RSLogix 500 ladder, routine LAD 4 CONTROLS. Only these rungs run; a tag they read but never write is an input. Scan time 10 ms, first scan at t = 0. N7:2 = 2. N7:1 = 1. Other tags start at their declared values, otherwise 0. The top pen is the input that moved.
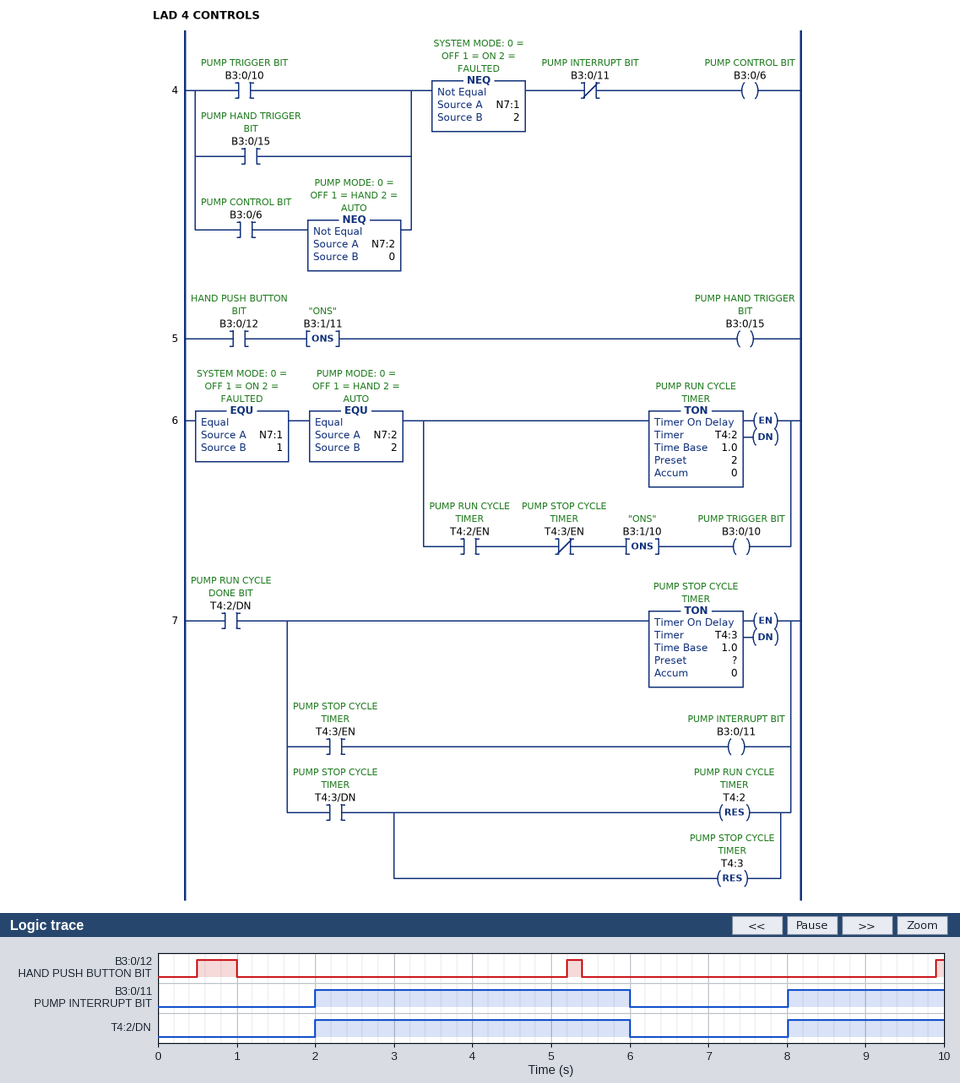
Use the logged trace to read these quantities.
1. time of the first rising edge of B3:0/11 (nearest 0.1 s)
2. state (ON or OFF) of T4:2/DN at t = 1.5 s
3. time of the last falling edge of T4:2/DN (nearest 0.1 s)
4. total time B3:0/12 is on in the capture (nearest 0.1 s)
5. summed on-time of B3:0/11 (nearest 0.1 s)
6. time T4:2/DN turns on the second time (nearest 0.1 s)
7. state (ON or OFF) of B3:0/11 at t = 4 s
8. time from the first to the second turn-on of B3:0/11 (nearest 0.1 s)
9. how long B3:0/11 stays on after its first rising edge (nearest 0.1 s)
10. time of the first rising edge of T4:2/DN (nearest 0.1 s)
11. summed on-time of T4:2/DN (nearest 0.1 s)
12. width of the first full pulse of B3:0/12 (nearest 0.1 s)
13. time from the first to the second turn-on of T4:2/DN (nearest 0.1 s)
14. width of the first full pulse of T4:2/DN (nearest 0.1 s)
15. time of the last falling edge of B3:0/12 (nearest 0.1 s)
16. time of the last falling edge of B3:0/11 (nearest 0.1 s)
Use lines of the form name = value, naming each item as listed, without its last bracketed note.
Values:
time of the first rising edge of B3:0/11 = 2.0 s
state (ON or OFF) of T4:2/DN at t = 1.5 s = OFF
time of the last falling edge of T4:2/DN = 6.0 s
total time B3:0/12 is on in the capture = 0.8 s
summed on-time of B3:0/11 = 6.0 s
time T4:2/DN turns on the second time = 8.0 s
state (ON or OFF) of B3:0/11 at t = 4 s = ON
time from the first to the second turn-on of B3:0/11 = 6.0 s
how long B3:0/11 stays on after its first rising edge = 4.0 s
time of the first rising edge of T4:2/DN = 2.0 s
summed on-time of T4:2/DN = 6.0 s
width of the first full pulse of B3:0/12 = 0.5 s
time from the first to the second turn-on of T4:2/DN = 6.0 s
width of the first full pulse of T4:2/DN = 4.0 s
time of the last falling edge of B3:0/12 = 5.4 s
time of the last falling edge of B3:0/11 = 6.0 s
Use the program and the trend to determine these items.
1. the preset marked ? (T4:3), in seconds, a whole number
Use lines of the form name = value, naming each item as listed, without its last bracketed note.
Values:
the preset marked ? (T4:3), in seconds, a whole number = 4 s
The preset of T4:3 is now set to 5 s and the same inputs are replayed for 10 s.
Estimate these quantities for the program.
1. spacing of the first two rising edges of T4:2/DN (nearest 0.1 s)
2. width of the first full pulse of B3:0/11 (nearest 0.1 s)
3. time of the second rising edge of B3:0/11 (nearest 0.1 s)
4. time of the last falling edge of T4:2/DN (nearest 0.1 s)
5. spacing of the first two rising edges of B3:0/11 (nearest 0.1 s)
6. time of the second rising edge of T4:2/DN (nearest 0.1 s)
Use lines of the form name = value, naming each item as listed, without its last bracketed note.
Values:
spacing of the first two rising edges of T4:2/DN = 7.0 s
width of the first full pulse of B3:0/11 = 5.0 s
time of the second rising edge of B3:0/11 = 9.0 s
time of the last falling edge of T4:2/DN = 7.0 s
spacing of the first two rising edges of B3:0/11 = 7.0 s
time of the second rising edge of T4:2/DN = 9.0 s
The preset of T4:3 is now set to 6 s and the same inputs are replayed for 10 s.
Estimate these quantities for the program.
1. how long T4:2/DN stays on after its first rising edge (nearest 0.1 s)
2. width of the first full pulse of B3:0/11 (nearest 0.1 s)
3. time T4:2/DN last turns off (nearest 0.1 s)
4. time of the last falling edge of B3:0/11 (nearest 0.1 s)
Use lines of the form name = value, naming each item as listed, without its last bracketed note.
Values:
how long T4:2/DN stays on after its first rising edge = 6.0 s
width of the first full pulse of B3:0/11 = 6.0 s
time T4:2/DN last turns off = 8.0 s
time of the last falling edge of B3:0/11 = 8.0 s
